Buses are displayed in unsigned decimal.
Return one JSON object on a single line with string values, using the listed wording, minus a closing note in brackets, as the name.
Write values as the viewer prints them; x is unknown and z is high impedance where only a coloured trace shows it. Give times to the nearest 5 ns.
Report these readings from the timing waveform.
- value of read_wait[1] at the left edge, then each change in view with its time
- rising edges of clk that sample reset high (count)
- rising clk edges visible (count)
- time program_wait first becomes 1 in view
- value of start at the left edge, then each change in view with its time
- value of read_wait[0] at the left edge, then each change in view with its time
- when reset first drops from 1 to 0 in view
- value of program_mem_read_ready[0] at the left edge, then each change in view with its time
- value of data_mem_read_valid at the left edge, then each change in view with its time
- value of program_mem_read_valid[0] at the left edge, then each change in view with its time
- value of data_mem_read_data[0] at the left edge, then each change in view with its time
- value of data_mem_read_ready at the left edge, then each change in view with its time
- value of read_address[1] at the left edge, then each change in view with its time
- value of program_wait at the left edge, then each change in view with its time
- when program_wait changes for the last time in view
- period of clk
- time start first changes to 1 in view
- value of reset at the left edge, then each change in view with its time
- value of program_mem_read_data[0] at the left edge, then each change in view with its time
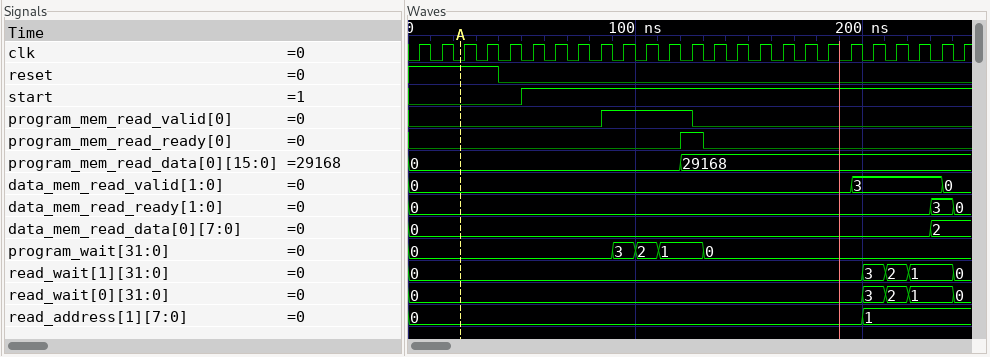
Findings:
{"value of read_wait[1] at the left edge, then each change in view with its time": "0, 3 at 200 ns, 2 at 210 ns, 1 at 220 ns, 0 at 240 ns", "rising edges of clk that sample reset high": "4", "rising clk edges visible": "25", "time program_wait first becomes 1 in view": "110 ns", "value of start at the left edge, then each change in view with its time": "0, 1 at 50 ns", "value of read_wait[0] at the left edge, then each change in view with its time": "0, 3 at 200 ns, 2 at 210 ns, 1 at 220 ns, 0 at 240 ns", "when reset first drops from 1 to 0 in view": "40 ns", "value of program_mem_read_ready[0] at the left edge, then each change in view with its time": "0, 1 at 120 ns, 0 at 130 ns", "value of data_mem_read_valid at the left edge, then each change in view with its time": "0, 3 at 195 ns, 0 at 235 ns", "value of program_mem_read_valid[0] at the left edge, then each change in view with its time": "0, 1 at 85 ns, 0 at 125 ns", "value of data_mem_read_data[0] at the left edge, then each change in view with its time": "0, 2 at 230 ns", "value of data_mem_read_ready at the left edge, then each change in view with its time": "0, 3 at 230 ns, 0 at 240 ns", "value of read_address[1] at the left edge, then each change in view with its time": "0, 1 at 200 ns", "value of program_wait at the left edge, then each change in view with its time": "0, 3 at 90 ns, 2 at 100 ns, 1 at 110 ns, 0 at 130 ns", "when program_wait changes for the last time in view": "130 ns", "period of clk": "10 ns", "time start first changes to 1 in view": "50 ns", "value of reset at the left edge, then each change in view with its time": "1, 0 at 40 ns", "value of program_mem_read_data[0] at the left edge, then each change in view with its time": "0, 29168 at 120 ns"}
